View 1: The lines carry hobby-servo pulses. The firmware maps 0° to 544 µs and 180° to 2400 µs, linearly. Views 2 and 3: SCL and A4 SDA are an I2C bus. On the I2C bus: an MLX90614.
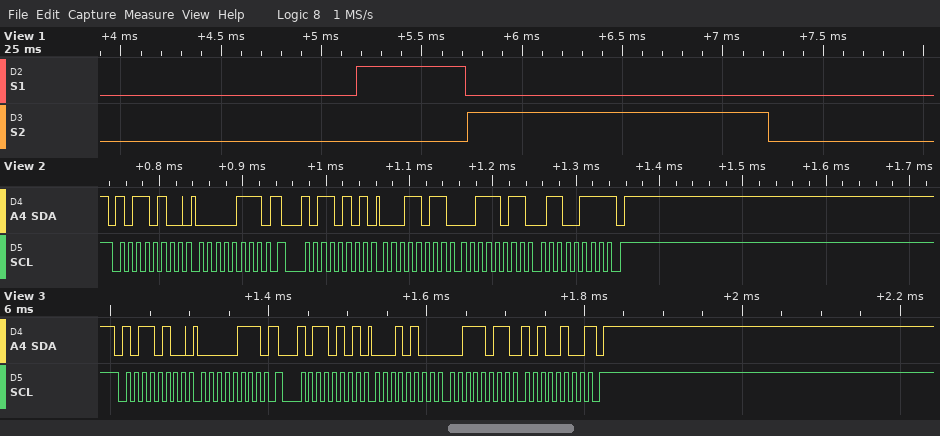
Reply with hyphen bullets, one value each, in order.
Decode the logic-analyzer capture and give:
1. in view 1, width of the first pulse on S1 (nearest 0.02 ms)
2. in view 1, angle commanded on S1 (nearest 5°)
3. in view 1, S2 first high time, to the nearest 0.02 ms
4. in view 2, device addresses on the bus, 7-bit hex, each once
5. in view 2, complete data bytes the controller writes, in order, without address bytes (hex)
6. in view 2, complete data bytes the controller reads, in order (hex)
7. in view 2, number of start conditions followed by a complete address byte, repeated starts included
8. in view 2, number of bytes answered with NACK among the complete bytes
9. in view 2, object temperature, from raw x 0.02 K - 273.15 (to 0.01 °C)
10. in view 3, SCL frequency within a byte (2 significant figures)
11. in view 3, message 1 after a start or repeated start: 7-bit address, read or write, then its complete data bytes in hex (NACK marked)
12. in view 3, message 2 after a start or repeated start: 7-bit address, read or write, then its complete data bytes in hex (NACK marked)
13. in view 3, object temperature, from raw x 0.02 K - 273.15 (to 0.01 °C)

- 0.54 ms
- 0°
- 1.50 ms
- 0x5A
- 07
- 1B 3B 67
- 2
- 1
- 29.47 °C
- 100 kHz
- 0x5A write: 07
- 0x5A read: 14 3B A4 NACK
- 29.33 °C
